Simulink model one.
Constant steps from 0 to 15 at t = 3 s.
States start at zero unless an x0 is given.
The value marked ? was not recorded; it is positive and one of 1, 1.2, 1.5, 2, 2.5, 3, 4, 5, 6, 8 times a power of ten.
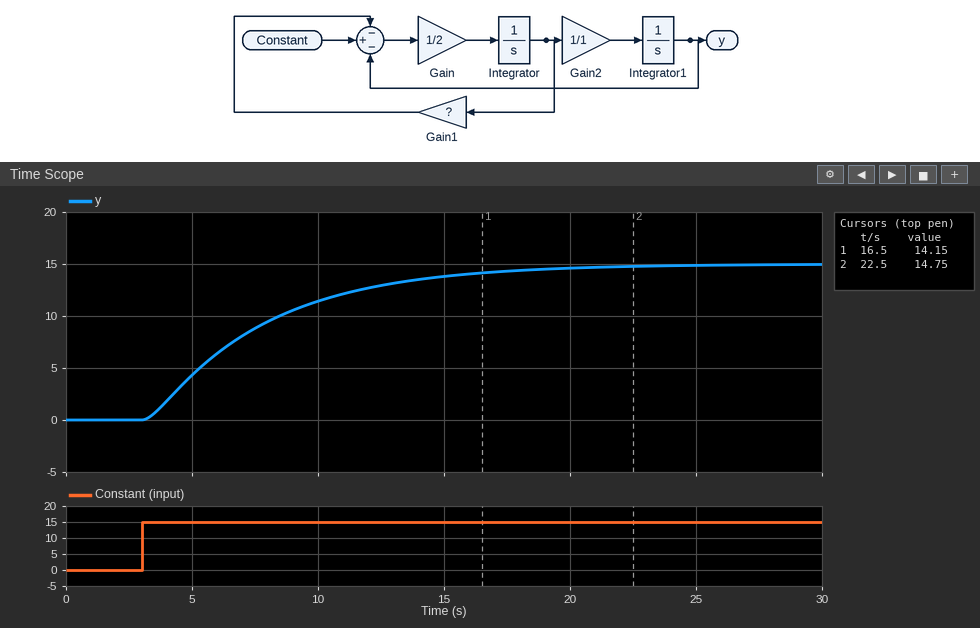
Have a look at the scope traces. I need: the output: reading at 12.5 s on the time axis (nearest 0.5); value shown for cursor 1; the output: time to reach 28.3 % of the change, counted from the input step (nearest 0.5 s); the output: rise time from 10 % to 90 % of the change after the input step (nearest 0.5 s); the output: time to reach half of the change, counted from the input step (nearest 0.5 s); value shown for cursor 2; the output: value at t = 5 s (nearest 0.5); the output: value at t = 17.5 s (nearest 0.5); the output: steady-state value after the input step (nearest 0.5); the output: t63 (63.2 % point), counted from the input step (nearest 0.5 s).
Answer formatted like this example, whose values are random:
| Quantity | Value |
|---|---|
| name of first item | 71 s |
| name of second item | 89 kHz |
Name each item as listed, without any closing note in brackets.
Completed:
| Quantity | Value |
|---|---|
| the output: reading at 12.5 s on the time axis | 13.0 |
| value shown for cursor 1 | 14.15 |
| the output: time to reach 28.3 % of the change, counted from the input step | 2.0 s |
| the output: rise time from 10 % to 90 % of the change after the input step | 10.0 s |
| the output: time to reach half of the change, counted from the input step | 3.5 s |
| value shown for cursor 2 | 14.75 |
| the output: value at t = 5 s | 4.5 |
| the output: value at t = 17.5 s | 14.5 |
| the output: steady-state value after the input step | 15.0 |
| the output: t63 (63.2 % point), counted from the input step | 5.0 s |
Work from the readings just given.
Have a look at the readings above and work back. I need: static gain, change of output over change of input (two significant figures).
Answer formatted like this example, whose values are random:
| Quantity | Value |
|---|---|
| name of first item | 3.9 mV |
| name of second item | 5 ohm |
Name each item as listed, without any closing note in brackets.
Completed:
| Quantity | Value |
|---|---|
| static gain, change of output over change of input | 1.0 |
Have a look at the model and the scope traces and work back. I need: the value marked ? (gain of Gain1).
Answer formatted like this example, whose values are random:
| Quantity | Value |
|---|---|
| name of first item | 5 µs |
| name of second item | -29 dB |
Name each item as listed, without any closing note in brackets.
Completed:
| Quantity | Value |
|---|---|
| the value marked ? | 5 |
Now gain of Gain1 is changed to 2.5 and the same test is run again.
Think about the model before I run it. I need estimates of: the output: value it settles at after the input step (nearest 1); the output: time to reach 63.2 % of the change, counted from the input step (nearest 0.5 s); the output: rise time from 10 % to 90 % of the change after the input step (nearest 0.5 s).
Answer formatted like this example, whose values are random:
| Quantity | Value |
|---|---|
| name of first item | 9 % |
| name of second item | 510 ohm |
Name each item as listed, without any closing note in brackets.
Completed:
| Quantity | Value |
|---|---|
| the output: value it settles at after the input step | 15 |
| the output: time to reach 63.2 % of the change, counted from the input step | 3.0 s |
| the output: rise time from 10 % to 90 % of the change after the input step | 4.0 s |
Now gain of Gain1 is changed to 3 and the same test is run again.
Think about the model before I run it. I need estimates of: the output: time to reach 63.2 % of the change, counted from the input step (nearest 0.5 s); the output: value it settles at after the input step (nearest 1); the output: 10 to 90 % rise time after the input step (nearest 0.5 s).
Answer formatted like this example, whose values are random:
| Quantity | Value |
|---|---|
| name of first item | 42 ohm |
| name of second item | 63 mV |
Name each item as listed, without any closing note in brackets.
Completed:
| Quantity | Value |
|---|---|
| the output: time to reach 63.2 % of the change, counted from the input step | 3.0 s |
| the output: value it settles at after the input step | 15 |
| the output: 10 to 90 % rise time after the input step | 5.0 s |
